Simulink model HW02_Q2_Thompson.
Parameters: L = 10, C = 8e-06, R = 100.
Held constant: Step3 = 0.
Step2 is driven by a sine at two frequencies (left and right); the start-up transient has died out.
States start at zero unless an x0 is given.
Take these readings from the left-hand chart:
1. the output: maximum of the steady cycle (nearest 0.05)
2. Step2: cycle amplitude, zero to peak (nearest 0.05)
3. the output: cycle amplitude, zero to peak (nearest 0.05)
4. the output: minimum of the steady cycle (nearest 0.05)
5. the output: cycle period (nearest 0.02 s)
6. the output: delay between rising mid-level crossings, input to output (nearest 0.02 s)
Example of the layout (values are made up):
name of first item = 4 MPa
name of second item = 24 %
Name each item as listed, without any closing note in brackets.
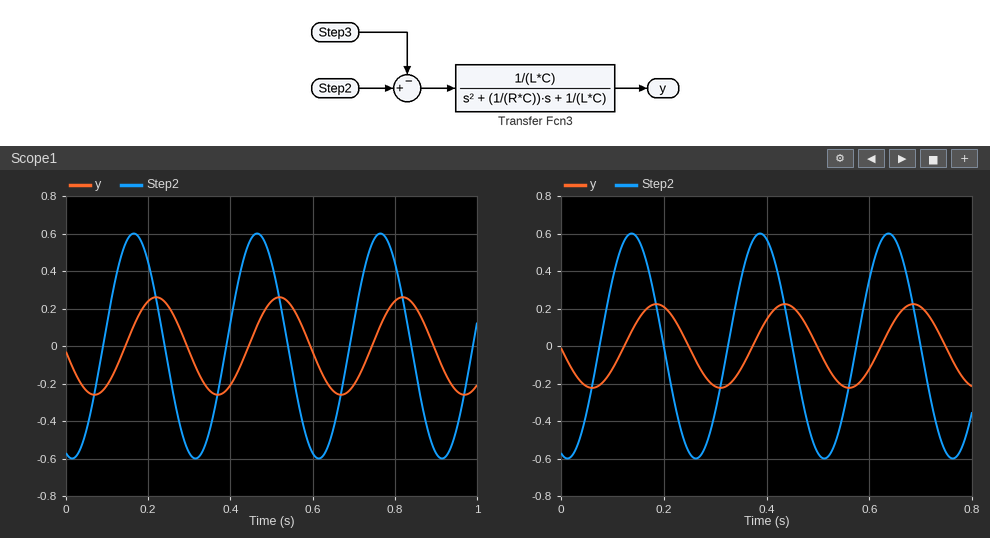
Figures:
the output: maximum of the steady cycle = 0.25
Step2: cycle amplitude, zero to peak = 0.60
the output: cycle amplitude, zero to peak = 0.25
the output: minimum of the steady cycle = -0.25
the output: cycle period = 0.30 s
the output: delay between rising mid-level crossings, input to output = 0.06 s
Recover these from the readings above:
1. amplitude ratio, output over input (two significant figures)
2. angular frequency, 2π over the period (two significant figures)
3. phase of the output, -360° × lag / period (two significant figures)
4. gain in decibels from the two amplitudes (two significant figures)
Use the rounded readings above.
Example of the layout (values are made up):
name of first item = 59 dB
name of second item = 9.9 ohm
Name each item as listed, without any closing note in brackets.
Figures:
amplitude ratio, output over input = 0.42
angular frequency, 2π over the period = 21 rad/s
phase of the output, -360° × lag / period = -72°
gain in decibels from the two amplitudes = -7.6 dB
